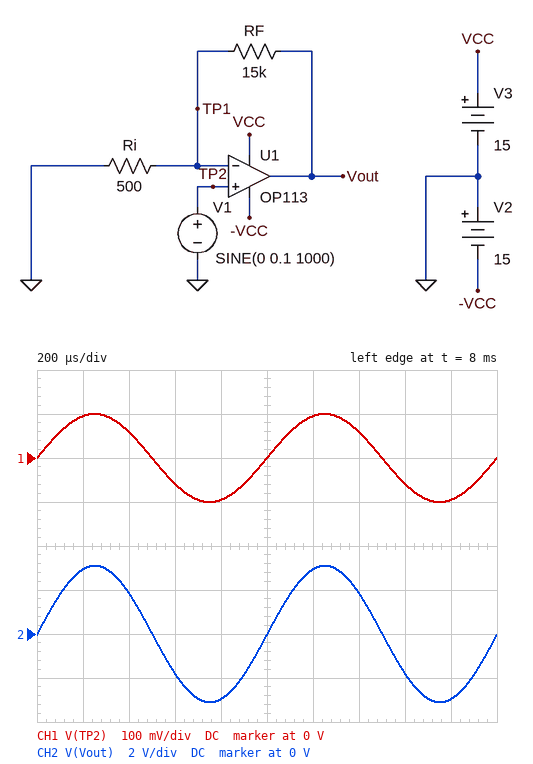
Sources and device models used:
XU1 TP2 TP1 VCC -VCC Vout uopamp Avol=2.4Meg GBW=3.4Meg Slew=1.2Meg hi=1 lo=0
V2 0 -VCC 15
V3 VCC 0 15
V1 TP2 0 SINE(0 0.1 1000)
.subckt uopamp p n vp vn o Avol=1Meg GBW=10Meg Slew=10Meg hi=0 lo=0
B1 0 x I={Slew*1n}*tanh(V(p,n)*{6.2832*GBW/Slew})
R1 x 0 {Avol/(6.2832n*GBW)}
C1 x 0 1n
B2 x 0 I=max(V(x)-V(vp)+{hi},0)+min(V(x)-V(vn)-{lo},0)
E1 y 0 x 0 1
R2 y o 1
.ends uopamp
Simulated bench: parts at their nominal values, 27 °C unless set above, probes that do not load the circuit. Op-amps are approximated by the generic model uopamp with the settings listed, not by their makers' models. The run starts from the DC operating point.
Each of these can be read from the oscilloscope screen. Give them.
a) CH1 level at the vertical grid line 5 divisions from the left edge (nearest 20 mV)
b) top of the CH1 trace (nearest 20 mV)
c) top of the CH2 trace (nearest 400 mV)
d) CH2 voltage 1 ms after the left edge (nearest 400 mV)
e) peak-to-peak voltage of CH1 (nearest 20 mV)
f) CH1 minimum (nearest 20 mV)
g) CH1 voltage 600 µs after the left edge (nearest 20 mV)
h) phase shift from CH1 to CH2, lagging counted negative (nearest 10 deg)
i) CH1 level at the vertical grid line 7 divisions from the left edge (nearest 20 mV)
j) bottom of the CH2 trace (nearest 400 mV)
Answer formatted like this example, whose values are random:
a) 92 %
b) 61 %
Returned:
a) 0 V
b) 100 mV
c) 3.2 V
d) 0 V
e) 200 mV
f) -100 mV
g) -60 mV
h) 0 deg
i) 60 mV
j) -3.2 V
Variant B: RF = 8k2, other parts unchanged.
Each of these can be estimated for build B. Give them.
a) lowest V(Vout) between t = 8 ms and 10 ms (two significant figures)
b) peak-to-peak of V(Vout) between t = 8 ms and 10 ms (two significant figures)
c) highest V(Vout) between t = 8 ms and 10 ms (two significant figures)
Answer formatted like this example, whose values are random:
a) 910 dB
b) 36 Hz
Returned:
a) -1.7 V
b) 3.5 V
c) 1.7 V
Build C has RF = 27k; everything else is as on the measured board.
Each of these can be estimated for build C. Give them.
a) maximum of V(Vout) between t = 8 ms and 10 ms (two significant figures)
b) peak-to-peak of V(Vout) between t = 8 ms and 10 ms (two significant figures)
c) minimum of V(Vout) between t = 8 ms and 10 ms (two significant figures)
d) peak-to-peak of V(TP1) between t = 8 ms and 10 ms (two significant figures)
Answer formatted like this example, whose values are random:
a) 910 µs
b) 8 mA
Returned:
a) 5.5 V
b) 11 V
c) -5.5 V
d) 200 mV
